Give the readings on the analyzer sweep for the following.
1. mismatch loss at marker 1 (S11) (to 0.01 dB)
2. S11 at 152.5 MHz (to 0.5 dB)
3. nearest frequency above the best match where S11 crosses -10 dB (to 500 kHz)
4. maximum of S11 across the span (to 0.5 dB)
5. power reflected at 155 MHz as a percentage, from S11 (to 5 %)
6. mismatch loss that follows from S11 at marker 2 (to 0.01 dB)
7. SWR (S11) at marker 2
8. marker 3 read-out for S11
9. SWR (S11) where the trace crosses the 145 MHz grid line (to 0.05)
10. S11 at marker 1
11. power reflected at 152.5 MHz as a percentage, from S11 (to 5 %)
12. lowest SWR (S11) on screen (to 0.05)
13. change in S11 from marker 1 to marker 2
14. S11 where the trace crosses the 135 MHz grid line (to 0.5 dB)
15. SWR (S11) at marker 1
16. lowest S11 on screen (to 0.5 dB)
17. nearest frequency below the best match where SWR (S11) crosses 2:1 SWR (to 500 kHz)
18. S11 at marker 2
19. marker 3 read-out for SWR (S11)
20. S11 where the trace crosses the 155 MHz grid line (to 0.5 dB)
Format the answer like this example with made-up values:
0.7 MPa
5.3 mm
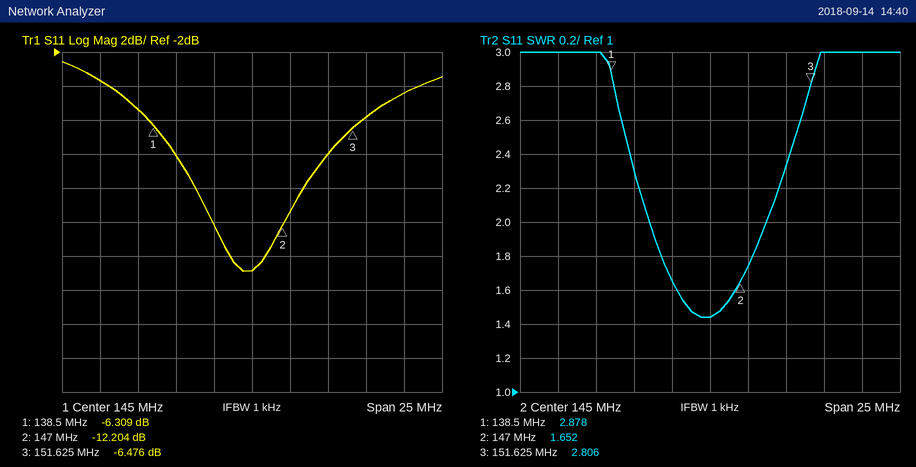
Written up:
1.16 dB
-6.0 dB
148.5 MHz
-2.5 dB
35 %
0.27 dB
1.652
-6.476 dB
1.45
-6.309 dB
25 %
1.45
-5.895 dB
-3.5 dB
2.878
-15.0 dB
141.0 MHz
-12.204 dB
2.806
-4.5 dB
